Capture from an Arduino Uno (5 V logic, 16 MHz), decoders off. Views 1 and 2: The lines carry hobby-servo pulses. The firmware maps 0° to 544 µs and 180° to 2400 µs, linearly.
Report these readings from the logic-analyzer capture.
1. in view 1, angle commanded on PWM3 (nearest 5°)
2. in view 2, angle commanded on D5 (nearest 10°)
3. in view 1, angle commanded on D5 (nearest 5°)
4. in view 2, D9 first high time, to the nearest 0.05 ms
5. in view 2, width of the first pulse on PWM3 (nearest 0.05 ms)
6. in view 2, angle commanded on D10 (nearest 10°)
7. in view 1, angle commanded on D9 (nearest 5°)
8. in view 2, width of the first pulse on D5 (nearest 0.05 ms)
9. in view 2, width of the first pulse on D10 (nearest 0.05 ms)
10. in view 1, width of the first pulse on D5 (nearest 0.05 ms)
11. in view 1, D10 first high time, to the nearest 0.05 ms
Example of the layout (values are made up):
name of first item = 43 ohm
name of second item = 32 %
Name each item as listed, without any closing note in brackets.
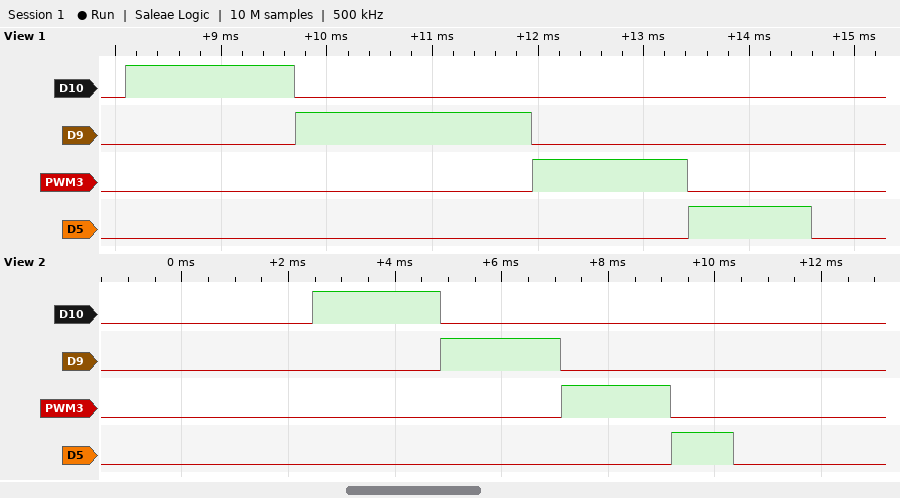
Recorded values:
in view 1, angle commanded on PWM3 = 90°
in view 2, angle commanded on D5 = 60°
in view 1, angle commanded on D5 = 60°
in view 2, D9 first high time, to the nearest 0.05 ms = 2.25 ms
in view 2, width of the first pulse on PWM3 = 2.05 ms
in view 2, angle commanded on D10 = 180°
in view 1, angle commanded on D9 = 165°
in view 2, width of the first pulse on D5 = 1.15 ms
in view 2, width of the first pulse on D10 = 2.40 ms
in view 1, width of the first pulse on D5 = 1.15 ms
in view 1, D10 first high time, to the nearest 0.05 ms = 1.60 ms
